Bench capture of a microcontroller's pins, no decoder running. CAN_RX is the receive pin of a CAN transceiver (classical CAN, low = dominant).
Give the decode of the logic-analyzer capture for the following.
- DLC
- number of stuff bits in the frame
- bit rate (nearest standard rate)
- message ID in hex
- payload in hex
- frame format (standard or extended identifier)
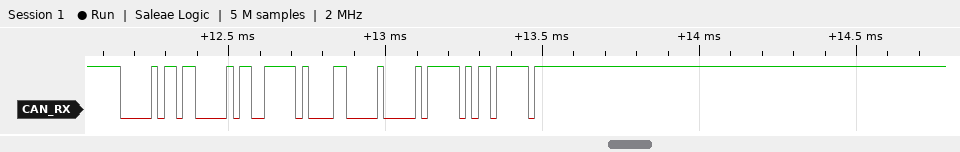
3
6
50 kbit/s
0x036
3F 0C 00
standard
